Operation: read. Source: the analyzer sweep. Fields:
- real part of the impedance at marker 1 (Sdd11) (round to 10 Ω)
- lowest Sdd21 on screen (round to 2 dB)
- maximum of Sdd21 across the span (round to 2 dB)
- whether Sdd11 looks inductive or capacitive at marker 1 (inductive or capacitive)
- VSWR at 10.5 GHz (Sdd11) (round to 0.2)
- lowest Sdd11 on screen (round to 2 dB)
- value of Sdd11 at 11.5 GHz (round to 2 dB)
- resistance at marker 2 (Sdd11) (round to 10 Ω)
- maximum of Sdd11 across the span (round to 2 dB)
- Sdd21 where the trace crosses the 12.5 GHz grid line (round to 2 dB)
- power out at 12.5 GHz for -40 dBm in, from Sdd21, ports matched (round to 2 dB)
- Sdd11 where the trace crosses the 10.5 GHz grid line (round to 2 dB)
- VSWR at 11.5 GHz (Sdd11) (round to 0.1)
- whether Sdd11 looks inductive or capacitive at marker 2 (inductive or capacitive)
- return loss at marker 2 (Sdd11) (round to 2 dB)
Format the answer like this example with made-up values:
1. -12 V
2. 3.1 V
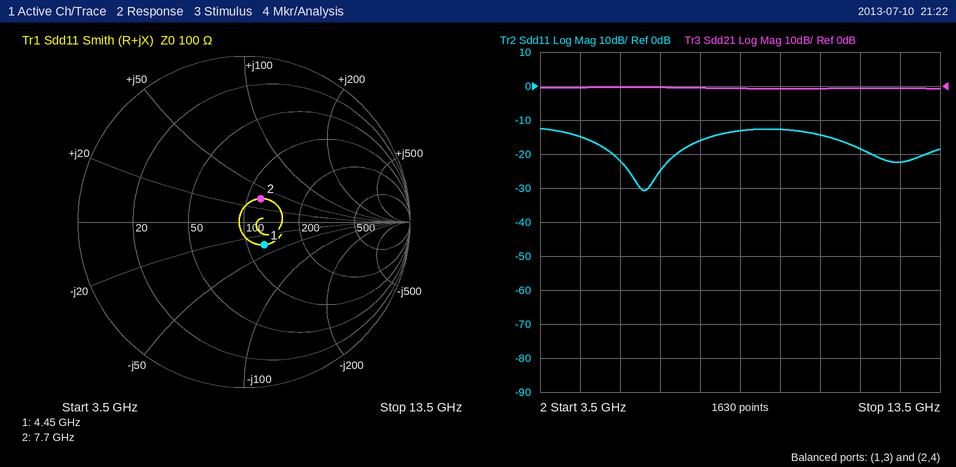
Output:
1. 120 Ω
2. 0 dB
3. 0 dB
4. capacitive
5. 1.4
6. -30 dB
7. -18 dB
8. 120 Ω
9. -12 dB
10. 0 dB
11. -40 dBm
12. -14 dB
13. 1.3
14. inductive
15. 16 dB
